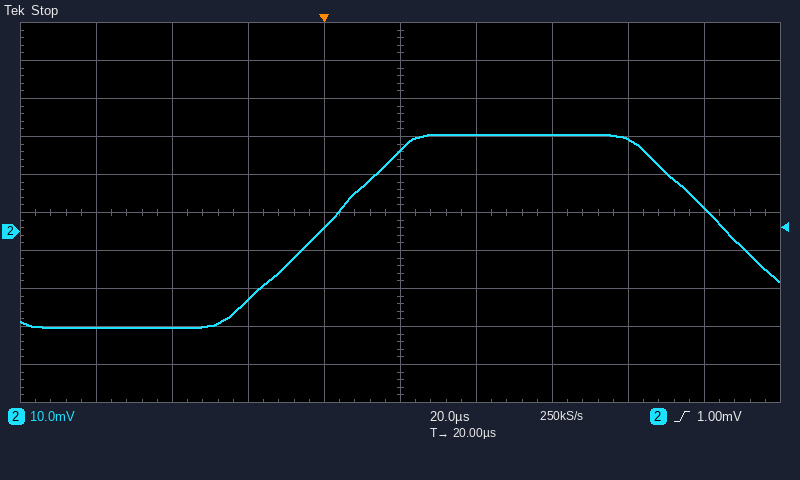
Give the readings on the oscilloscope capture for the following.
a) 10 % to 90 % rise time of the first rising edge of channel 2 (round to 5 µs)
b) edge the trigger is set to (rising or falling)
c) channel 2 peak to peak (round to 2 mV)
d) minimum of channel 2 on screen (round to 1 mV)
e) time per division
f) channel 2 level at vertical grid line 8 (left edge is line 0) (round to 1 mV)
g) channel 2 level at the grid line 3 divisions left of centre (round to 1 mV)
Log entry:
40 µs
rising
50 mV
-25 mV
20 µs
24 mV
-25 mV
